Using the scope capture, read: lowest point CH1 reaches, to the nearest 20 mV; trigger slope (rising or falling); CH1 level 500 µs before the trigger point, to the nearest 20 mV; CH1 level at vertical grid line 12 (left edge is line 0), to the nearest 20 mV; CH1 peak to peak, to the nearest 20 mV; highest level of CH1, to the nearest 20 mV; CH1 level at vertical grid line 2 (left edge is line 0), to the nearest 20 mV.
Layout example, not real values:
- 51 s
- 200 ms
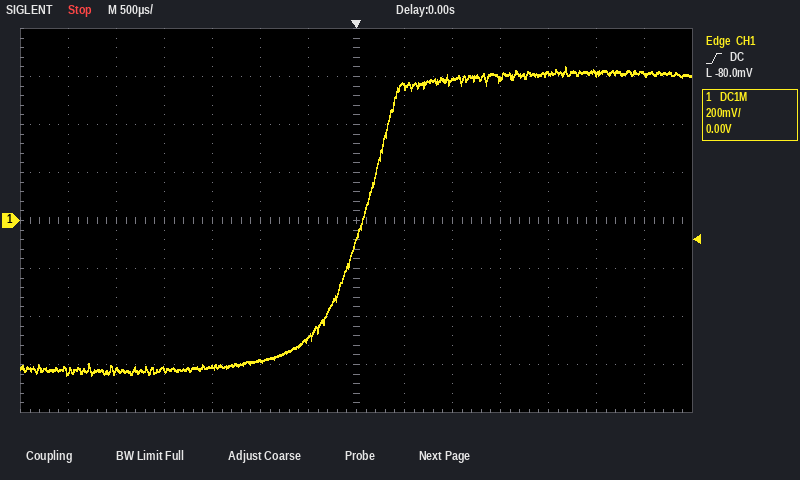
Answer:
- -640 mV
- rising
- -500 mV
- 620 mV
- 1.28 V
- 640 mV
- -620 mV
